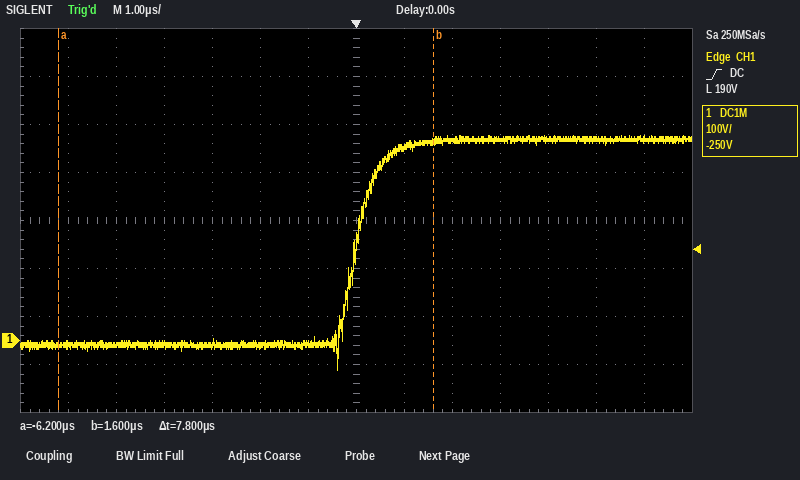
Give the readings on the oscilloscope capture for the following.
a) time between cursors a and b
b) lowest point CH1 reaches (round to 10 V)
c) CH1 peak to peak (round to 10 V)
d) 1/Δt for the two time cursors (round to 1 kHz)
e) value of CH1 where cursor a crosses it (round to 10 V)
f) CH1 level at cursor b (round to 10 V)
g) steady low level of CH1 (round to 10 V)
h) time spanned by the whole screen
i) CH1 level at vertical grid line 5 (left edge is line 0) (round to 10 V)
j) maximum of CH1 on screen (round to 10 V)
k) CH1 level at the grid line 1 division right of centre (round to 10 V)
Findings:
7.8 µs
-60 V
490 V
128 kHz
-10 V
420 V
-10 V
14 µs
-10 V
430 V
400 V
